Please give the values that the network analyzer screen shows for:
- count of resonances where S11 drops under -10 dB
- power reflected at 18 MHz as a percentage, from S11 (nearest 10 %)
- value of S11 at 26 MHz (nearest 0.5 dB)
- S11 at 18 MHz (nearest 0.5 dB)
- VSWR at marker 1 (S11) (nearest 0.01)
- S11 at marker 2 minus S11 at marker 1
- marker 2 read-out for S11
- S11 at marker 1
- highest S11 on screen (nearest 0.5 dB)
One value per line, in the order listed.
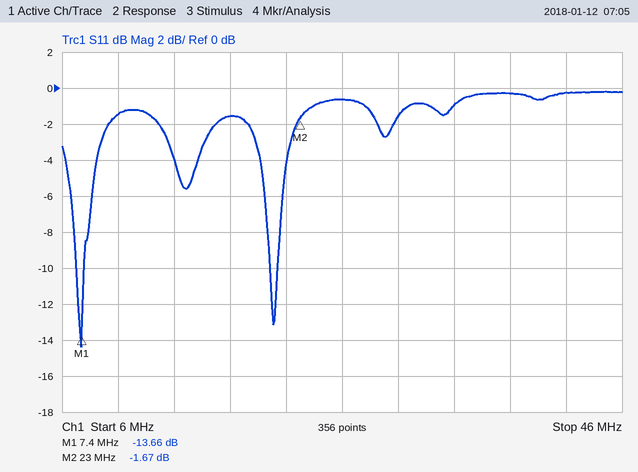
2
70 %
-0.5 dB
-1.5 dB
1.52
11.99 dB
-1.67 dB
-13.66 dB
0.0 dB
